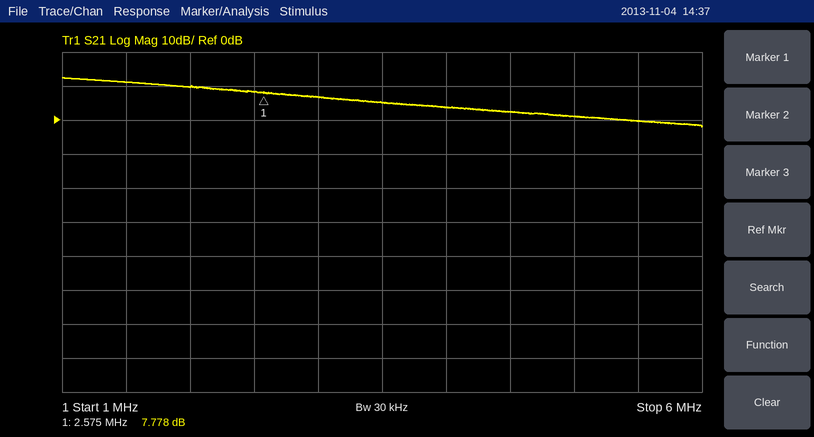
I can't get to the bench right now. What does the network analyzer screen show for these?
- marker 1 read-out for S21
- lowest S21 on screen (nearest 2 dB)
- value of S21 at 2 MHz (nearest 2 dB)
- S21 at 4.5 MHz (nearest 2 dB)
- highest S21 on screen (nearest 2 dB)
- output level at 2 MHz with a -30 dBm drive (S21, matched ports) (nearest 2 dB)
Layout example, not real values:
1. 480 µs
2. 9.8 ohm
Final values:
1. 7.778 dB
2. -2 dB
3. 10 dB
4. 2 dB
5. 12 dB
6. -20 dBm
